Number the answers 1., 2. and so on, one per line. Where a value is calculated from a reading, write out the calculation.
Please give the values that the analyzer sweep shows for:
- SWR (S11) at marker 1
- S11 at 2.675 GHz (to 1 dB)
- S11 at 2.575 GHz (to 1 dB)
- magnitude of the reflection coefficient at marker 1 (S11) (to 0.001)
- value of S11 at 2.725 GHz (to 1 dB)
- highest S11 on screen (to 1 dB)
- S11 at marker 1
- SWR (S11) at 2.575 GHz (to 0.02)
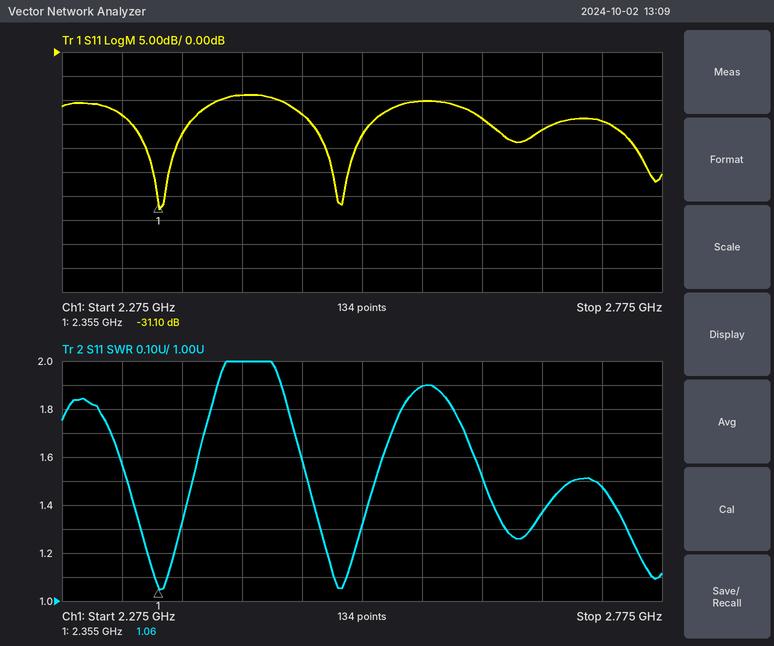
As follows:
1. 1.06
2. -16 dB
3. -10 dB
4. 10^(-31.1/20) ≈ 0.028
5. -14 dB
6. -9 dB
7. -31.10 dB
8. 1.90
